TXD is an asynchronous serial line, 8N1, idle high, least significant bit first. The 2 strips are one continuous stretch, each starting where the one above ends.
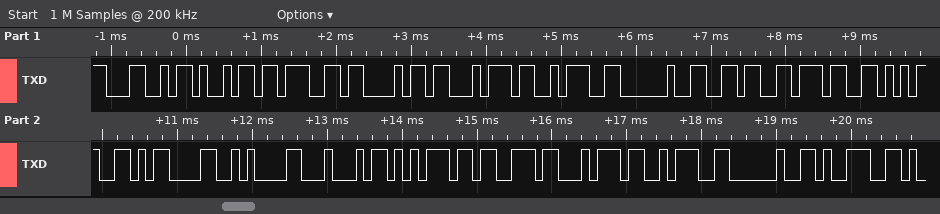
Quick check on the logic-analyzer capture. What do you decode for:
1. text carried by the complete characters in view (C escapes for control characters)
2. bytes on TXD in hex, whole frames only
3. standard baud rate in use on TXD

"Light: 675\r\nDust: 9"
4C 69 67 68 74 3A 20 36 37 35 0D 0A 44 75 73 74 3A 20 39
9600 baud
